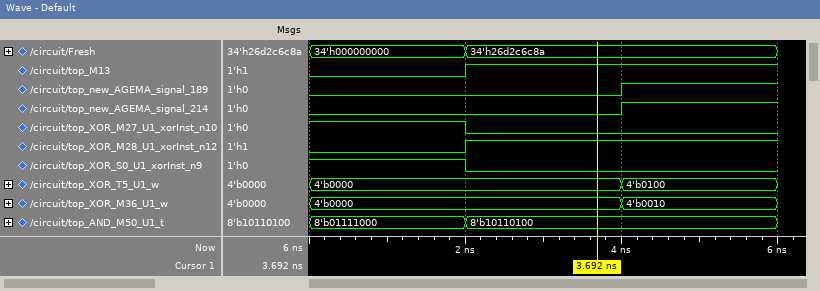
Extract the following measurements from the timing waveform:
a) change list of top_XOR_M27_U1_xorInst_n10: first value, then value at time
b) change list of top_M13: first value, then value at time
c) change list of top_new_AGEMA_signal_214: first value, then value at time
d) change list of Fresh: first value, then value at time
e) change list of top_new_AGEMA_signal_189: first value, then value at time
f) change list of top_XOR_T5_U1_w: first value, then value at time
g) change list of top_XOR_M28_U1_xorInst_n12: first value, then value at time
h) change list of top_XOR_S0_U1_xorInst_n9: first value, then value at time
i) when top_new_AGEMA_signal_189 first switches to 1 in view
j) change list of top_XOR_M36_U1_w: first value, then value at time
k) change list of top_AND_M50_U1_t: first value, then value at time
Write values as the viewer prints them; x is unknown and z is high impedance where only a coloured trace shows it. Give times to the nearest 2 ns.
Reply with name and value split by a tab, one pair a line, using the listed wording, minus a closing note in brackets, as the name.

change list of top_XOR_M27_U1_xorInst_n10: first value, then value at time	1, 0 at 2 ns
change list of top_M13: first value, then value at time	0, 1 at 2 ns
change list of top_new_AGEMA_signal_214: first value, then value at time	0, 1 at 4 ns
change list of Fresh: first value, then value at time	34'h000000000, 34'h26d2c6c8a at 2 ns
change list of top_new_AGEMA_signal_189: first value, then value at time	0, 1 at 4 ns
change list of top_XOR_T5_U1_w: first value, then value at time	4'b0000, 4'b0100 at 4 ns
change list of top_XOR_M28_U1_xorInst_n12: first value, then value at time	0, 1 at 2 ns
change list of top_XOR_S0_U1_xorInst_n9: first value, then value at time	1, 0 at 2 ns
when top_new_AGEMA_signal_189 first switches to 1 in view	4 ns
change list of top_XOR_M36_U1_w: first value, then value at time	4'b0000, 4'b0010 at 4 ns
change list of top_AND_M50_U1_t: first value, then value at time	8'b01111000, 8'b10110100 at 2 ns
